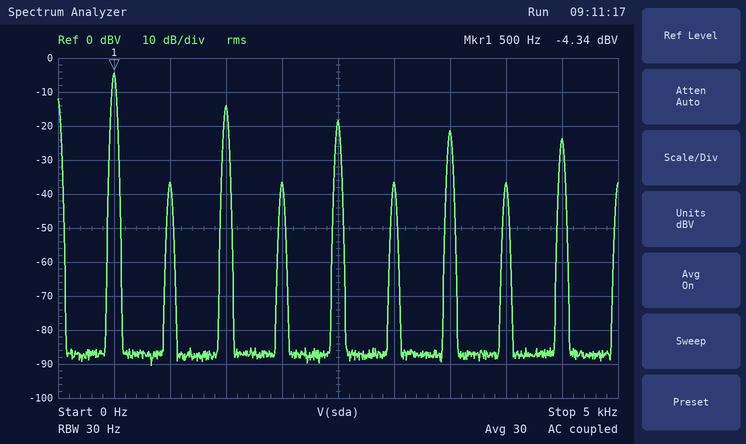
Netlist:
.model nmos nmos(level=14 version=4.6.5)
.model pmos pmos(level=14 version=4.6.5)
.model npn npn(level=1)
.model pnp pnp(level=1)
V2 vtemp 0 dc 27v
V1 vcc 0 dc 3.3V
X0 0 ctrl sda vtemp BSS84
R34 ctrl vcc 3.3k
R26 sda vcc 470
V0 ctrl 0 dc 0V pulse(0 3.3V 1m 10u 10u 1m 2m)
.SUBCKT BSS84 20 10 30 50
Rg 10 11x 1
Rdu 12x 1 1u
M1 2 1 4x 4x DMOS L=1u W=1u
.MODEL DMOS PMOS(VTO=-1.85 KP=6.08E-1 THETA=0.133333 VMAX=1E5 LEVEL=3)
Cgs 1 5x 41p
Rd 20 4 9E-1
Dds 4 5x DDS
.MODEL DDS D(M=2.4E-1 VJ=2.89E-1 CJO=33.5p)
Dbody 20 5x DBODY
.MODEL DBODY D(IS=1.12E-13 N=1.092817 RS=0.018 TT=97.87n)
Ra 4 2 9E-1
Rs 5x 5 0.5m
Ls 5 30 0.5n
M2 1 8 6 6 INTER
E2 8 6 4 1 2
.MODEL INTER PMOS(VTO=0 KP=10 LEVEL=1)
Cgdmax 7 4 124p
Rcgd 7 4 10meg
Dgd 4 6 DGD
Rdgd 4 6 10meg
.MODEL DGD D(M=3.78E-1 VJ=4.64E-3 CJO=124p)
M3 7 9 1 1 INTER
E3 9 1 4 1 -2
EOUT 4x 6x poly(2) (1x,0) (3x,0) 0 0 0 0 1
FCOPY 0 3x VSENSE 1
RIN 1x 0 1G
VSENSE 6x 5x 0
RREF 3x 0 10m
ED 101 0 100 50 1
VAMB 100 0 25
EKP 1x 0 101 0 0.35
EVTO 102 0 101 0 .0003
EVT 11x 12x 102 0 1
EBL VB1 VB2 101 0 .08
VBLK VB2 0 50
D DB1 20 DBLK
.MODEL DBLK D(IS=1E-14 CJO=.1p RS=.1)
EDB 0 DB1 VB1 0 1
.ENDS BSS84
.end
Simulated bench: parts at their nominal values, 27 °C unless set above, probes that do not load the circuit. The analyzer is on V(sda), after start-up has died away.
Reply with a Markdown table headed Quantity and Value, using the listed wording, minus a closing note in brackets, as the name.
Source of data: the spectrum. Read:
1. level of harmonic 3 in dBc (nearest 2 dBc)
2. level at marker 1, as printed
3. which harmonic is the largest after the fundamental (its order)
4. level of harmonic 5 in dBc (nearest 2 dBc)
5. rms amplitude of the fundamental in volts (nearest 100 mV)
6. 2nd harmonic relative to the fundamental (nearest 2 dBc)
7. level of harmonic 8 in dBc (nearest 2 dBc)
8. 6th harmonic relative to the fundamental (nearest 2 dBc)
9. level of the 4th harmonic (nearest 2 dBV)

| Quantity | Value |
|---|---|
| level of harmonic 3 in dBc | -10 dBc |
| level at marker 1, as printed | -4.34 dBV |
| which harmonic is the largest after the fundamental | 3 |
| level of harmonic 5 in dBc | -14 dBc |
| rms amplitude of the fundamental in volts | 600 mV |
| 2nd harmonic relative to the fundamental | -32 dBc |
| level of harmonic 8 in dBc | -32 dBc |
| 6th harmonic relative to the fundamental | -32 dBc |
| level of the 4th harmonic | -36 dBV |
